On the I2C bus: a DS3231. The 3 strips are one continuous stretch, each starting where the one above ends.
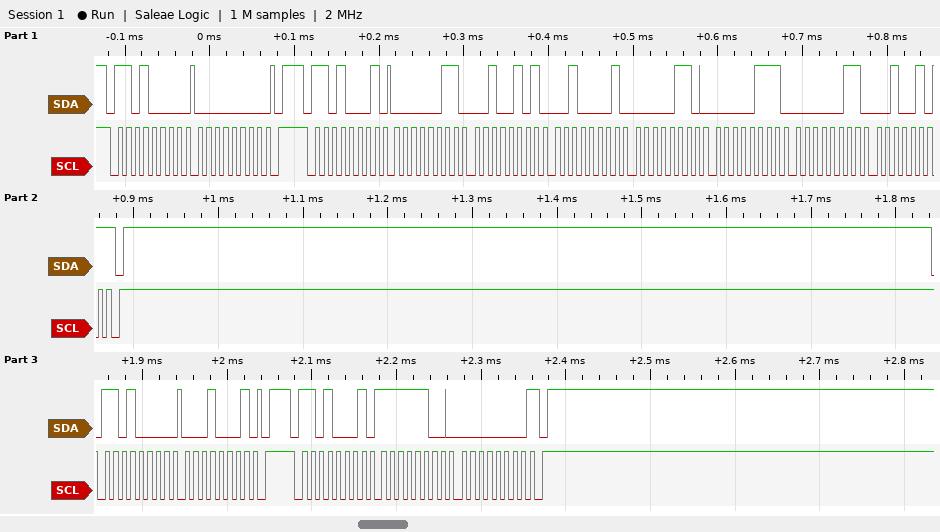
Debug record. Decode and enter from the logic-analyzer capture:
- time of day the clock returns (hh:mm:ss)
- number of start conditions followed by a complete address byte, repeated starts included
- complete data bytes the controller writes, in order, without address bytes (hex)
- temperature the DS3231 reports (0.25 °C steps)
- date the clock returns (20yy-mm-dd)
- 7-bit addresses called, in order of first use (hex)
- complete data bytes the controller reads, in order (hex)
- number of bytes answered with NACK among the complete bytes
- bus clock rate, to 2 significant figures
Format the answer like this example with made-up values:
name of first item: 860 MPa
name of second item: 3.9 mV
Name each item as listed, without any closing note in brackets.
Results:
time of day the clock returns: 21:25:03
number of start conditions followed by a complete address byte, repeated starts included: 4
complete data bytes the controller writes, in order, without address bytes: 00 11
temperature the DS3231 reports: -4.00 °C
date the clock returns: 2025-03-07
7-bit addresses called, in order of first use: 0x68
complete data bytes the controller reads, in order: 03 25 21 06 07 03 25 FC 00
number of bytes answered with NACK among the complete bytes: 2
bus clock rate, to 2 significant figures: 100 kHz
